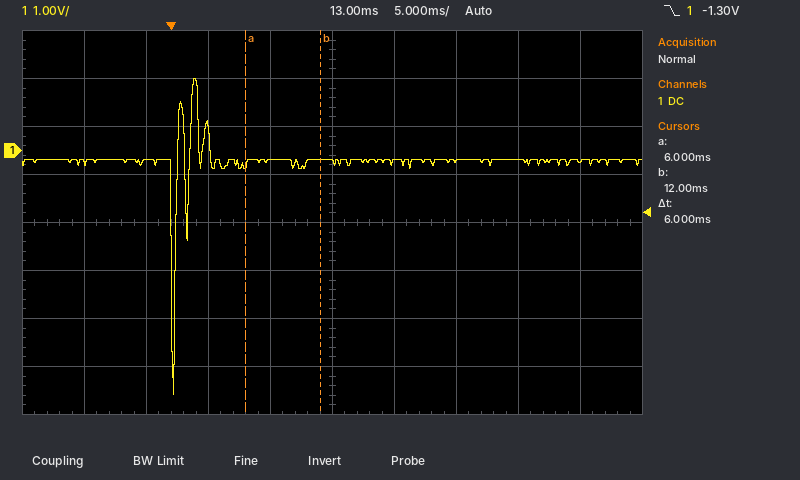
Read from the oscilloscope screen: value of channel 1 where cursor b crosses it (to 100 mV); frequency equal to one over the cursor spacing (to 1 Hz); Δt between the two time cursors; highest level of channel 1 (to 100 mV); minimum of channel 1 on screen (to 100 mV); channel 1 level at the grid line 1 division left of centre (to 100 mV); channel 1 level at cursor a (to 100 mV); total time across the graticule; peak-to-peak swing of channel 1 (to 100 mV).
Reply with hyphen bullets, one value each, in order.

- -200 mV
- 167 Hz
- 6 ms
- 1.5 V
- -5.1 V
- -200 mV
- -300 mV
- 50 ms
- 6.6 V
